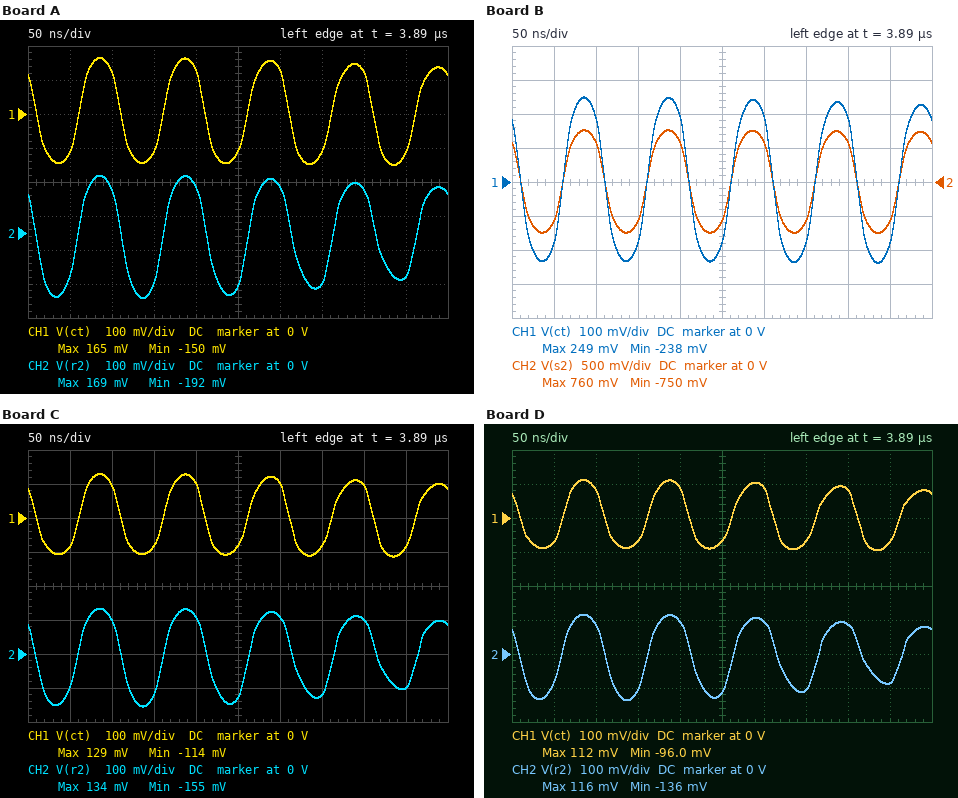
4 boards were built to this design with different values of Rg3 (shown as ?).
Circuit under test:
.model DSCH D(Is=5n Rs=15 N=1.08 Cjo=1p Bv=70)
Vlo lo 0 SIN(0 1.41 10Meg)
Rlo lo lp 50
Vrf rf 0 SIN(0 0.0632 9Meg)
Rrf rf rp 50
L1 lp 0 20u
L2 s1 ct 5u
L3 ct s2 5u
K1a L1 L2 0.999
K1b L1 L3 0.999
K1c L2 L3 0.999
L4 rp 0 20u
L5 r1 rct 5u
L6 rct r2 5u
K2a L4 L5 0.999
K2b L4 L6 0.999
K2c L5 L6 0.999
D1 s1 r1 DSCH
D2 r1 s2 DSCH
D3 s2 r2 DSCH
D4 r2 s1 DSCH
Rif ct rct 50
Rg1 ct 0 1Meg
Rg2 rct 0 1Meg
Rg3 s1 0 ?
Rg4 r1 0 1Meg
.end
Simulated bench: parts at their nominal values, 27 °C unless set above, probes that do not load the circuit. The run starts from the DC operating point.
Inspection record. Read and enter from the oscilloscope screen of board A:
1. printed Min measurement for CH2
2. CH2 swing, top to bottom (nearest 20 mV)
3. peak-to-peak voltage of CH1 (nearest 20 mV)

-192 mV
360 mV
320 mV
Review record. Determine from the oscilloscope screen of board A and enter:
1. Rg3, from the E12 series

820 kΩ
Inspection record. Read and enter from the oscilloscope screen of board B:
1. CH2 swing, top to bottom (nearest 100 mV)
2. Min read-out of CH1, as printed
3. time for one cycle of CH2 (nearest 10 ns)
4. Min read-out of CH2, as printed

1.5 V
-238 mV
100 ns
-750 mV
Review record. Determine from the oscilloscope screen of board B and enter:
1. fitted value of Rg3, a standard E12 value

390 kΩ
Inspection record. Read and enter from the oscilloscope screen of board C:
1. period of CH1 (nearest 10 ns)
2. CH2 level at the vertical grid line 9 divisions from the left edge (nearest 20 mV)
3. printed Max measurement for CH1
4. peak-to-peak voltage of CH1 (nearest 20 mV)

100 ns
-100 mV
129 mV
240 mV
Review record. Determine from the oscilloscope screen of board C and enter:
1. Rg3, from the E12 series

1.2 MΩ
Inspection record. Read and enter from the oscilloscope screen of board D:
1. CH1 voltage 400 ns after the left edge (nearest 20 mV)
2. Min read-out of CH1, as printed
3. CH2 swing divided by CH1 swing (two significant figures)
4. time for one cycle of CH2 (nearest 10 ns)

80 mV
-96.0 mV
1.2
100 ns
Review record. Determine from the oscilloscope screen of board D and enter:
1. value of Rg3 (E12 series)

1.5 MΩ
